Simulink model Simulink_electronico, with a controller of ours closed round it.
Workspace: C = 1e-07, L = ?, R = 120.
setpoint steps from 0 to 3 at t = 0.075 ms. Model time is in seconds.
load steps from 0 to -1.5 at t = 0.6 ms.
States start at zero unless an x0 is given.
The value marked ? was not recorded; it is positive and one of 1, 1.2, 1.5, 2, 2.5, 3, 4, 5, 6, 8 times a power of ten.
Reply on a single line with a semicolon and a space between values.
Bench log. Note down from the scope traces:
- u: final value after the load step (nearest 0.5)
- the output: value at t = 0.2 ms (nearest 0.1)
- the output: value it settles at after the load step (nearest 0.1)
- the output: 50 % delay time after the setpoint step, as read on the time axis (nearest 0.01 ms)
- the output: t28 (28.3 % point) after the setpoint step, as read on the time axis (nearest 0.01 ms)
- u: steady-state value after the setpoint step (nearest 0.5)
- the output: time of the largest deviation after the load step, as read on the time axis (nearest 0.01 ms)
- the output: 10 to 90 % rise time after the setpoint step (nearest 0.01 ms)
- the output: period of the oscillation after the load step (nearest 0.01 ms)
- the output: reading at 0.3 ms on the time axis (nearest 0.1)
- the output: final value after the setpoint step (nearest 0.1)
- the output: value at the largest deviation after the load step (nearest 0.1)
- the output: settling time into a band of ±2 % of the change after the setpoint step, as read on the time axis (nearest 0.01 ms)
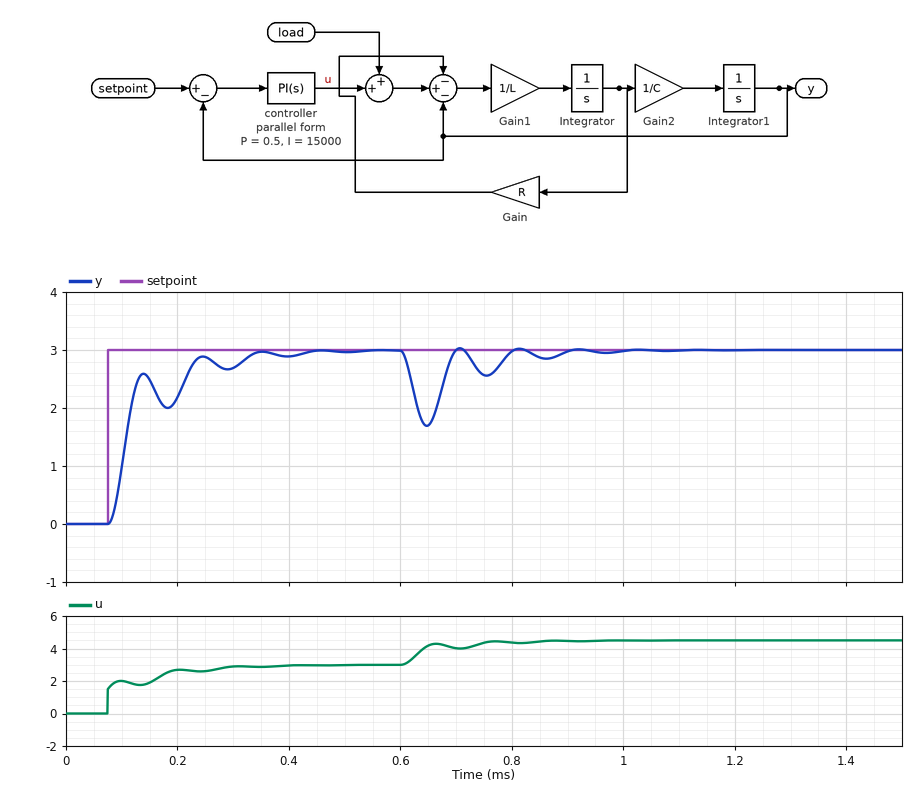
4.5; 2.2; 3.0; 0.11 ms; 0.10 ms; 3.0; 0.65 ms; 0.14 ms; 0.11 ms; 2.7; 3.0; 1.7; 0.43 ms
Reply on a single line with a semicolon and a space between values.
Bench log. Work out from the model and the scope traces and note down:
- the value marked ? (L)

0.004
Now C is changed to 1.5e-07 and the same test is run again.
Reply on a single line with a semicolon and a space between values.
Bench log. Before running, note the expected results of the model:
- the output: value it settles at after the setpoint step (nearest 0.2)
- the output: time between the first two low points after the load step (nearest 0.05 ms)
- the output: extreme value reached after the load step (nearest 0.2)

3.0; 0.15 ms; 1.8
